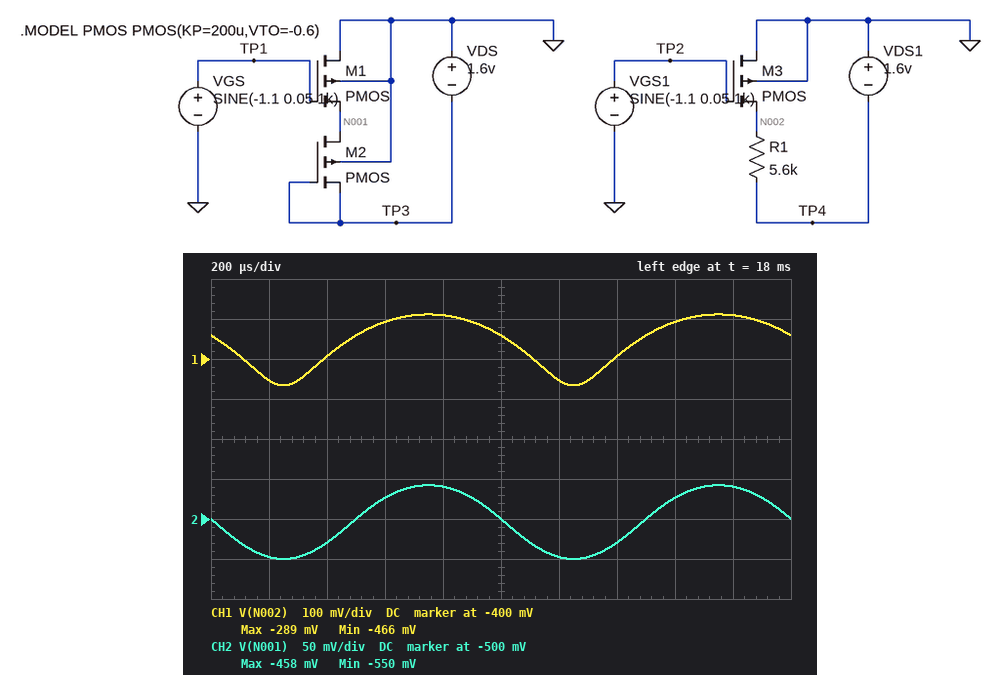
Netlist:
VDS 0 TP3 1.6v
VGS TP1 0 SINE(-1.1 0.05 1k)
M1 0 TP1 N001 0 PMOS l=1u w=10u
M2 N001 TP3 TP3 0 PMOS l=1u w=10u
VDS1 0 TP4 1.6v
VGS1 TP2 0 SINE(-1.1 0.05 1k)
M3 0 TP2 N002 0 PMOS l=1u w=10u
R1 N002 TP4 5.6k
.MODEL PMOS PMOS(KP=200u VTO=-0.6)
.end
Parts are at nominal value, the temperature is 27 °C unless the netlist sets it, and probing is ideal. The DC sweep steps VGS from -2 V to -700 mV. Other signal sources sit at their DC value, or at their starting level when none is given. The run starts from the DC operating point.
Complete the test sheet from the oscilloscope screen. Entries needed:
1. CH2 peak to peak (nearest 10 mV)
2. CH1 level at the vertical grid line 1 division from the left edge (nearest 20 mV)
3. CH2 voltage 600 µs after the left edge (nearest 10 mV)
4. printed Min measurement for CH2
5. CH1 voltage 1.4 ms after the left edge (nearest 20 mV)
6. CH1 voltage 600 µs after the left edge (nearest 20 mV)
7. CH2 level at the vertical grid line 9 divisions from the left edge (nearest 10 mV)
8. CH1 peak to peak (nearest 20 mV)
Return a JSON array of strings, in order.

["90 mV", "-460 mV", "-470 mV", "-550 mV", "-400 mV", "-300 mV", "-460 mV", "180 mV"]
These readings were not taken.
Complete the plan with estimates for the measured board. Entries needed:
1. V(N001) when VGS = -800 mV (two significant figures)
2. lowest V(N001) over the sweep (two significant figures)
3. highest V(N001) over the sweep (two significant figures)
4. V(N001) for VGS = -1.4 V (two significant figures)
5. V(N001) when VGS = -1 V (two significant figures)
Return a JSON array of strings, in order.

["-800 mV", "-900 mV", "-230 mV", "-340 mV", "-600 mV"]
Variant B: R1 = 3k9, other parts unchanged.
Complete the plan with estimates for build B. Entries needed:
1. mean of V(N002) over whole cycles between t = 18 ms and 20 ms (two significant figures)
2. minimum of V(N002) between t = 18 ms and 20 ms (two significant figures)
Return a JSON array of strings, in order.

["-630 mV", "-810 mV"]
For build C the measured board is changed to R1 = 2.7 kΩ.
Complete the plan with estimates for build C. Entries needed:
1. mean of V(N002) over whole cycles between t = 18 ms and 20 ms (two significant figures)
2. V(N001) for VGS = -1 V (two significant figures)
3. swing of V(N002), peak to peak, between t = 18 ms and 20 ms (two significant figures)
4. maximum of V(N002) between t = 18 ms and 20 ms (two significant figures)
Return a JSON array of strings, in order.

["-920 mV", "-600 mV", "270 mV", "-780 mV"]
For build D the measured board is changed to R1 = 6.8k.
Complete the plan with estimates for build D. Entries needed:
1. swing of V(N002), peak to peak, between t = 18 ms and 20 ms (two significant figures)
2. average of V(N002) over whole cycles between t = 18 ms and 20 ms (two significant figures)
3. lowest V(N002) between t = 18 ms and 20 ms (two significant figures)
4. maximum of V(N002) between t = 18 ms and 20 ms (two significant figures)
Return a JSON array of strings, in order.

["95 mV", "-270 mV", "-330 mV", "-230 mV"]
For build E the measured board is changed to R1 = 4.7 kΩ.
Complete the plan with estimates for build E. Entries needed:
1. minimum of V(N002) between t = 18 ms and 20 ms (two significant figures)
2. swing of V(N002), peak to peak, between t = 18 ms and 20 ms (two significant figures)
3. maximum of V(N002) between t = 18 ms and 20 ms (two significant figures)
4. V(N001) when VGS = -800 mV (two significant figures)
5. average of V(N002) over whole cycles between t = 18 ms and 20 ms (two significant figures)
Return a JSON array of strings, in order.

["-650 mV", "290 mV", "-360 mV", "-800 mV", "-480 mV"]
